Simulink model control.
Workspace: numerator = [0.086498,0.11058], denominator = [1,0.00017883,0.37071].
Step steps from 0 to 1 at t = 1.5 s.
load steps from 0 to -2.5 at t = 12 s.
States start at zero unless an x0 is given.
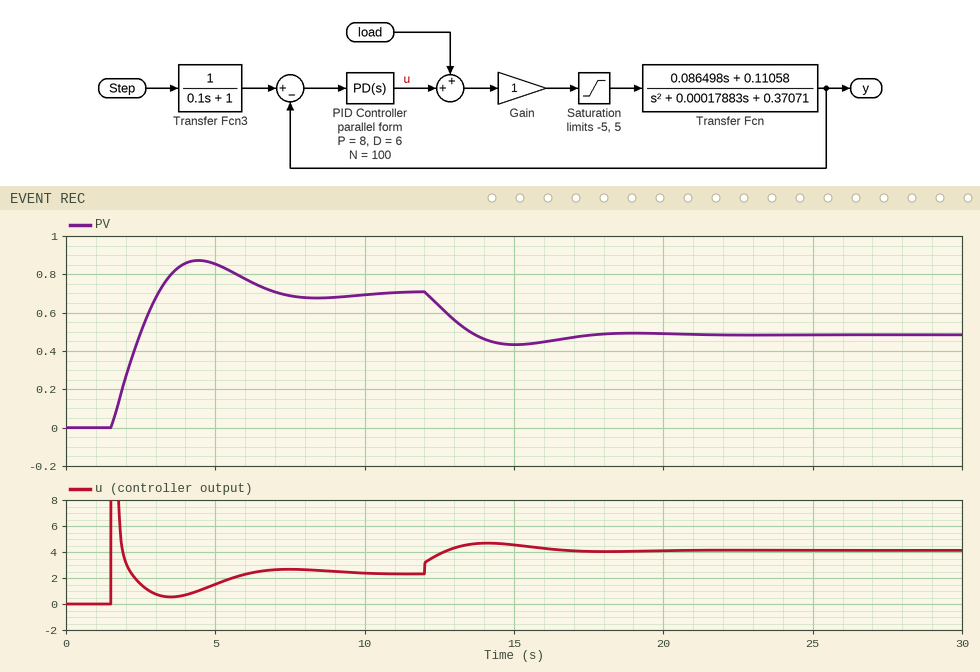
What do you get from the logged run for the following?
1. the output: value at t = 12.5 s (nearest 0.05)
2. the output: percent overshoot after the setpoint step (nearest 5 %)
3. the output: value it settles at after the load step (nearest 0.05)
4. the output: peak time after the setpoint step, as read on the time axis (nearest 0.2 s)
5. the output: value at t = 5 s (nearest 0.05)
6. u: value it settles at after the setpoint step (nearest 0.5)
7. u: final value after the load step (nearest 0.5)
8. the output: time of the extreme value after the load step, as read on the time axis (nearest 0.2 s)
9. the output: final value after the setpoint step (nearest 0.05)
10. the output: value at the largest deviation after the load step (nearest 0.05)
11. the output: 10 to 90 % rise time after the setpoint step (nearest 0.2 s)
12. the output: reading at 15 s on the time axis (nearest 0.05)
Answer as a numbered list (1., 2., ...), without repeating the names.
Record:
1. 0.65
2. 25 %
3. 0.50
4. 4.4 s
5. 0.85
6. 2.5
7. 4.0
8. 15.0 s
9. 0.70
10. 0.45
11. 1.2 s
12. 0.45
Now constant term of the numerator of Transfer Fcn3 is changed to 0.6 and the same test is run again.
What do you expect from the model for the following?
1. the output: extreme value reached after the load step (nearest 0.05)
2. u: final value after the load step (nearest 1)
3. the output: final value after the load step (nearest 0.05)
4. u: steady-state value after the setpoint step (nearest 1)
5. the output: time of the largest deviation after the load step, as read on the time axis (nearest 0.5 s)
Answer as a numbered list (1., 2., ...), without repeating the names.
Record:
1. 0.15
2. 3
3. 0.20
4. 1
5. 15.0 s
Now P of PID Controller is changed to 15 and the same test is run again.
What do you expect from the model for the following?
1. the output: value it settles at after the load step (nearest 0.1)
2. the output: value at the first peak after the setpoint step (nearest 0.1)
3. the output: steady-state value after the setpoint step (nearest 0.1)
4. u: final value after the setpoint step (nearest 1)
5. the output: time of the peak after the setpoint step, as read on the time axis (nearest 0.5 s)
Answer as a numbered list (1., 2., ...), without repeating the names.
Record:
1. 0.7
2. 1.0
3. 0.8
4. 3
5. 4.0 s
